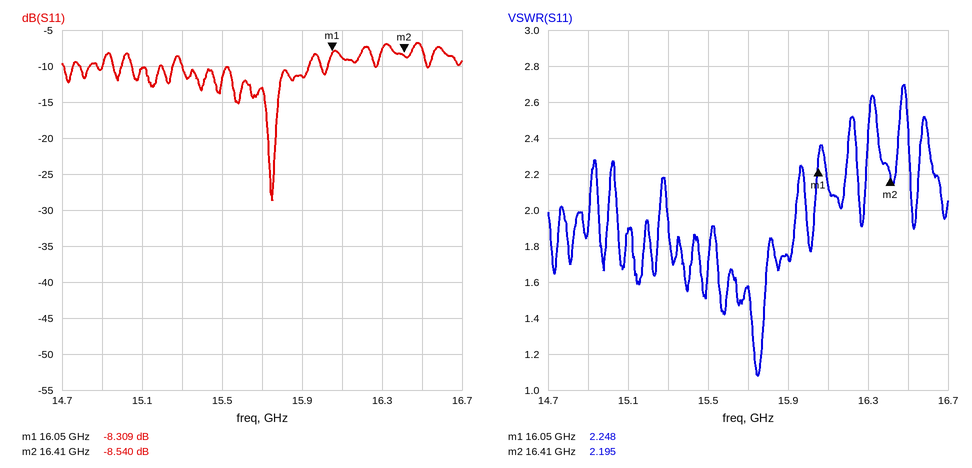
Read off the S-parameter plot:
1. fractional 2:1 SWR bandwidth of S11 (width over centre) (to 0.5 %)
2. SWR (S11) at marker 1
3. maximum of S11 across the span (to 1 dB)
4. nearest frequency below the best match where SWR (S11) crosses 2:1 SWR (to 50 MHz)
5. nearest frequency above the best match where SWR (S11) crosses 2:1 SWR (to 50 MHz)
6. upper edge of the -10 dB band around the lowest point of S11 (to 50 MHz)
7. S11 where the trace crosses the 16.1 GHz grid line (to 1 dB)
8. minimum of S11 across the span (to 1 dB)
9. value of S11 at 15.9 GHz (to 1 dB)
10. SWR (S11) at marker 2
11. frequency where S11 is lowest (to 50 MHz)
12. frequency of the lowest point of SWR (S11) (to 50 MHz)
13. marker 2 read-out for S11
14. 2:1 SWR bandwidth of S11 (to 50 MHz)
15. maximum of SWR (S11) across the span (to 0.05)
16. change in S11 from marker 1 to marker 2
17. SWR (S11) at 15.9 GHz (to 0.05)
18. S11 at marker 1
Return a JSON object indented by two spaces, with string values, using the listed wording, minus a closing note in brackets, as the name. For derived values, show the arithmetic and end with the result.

{
  "fractional 2:1 SWR bandwidth of S11 (width over centre)": "650 MHz / 15.625 GHz ≈ 4.16 %, so 4.0 % to the nearest 0.5 %",
  "SWR (S11) at marker 1": "2.248",
  "maximum of S11 across the span": "-7 dB",
  "nearest frequency below the best match where SWR (S11) crosses 2:1 SWR": "15.30 GHz",
  "nearest frequency above the best match where SWR (S11) crosses 2:1 SWR": "15.95 GHz",
  "upper edge of the -10 dB band around the lowest point of S11": "15.95 GHz",
  "S11 where the trace crosses the 16.1 GHz grid line": "-9 dB",
  "minimum of S11 across the span": "-29 dB",
  "value of S11 at 15.9 GHz": "-11 dB",
  "SWR (S11) at marker 2": "2.195",
  "frequency where S11 is lowest": "15.75 GHz",
  "frequency of the lowest point of SWR (S11)": "15.75 GHz",
  "marker 2 read-out for S11": "-8.540 dB",
  "2:1 SWR bandwidth of S11": "15.95 GHz − 15.30 GHz = 650 MHz",
  "maximum of SWR (S11) across the span": "2.70",
  "change in S11 from marker 1 to marker 2": "-8.54 − (-8.309) = -0.231 dB",
  "SWR (S11) at 15.9 GHz": "1.75",
  "S11 at marker 1": "-8.309 dB"
}
